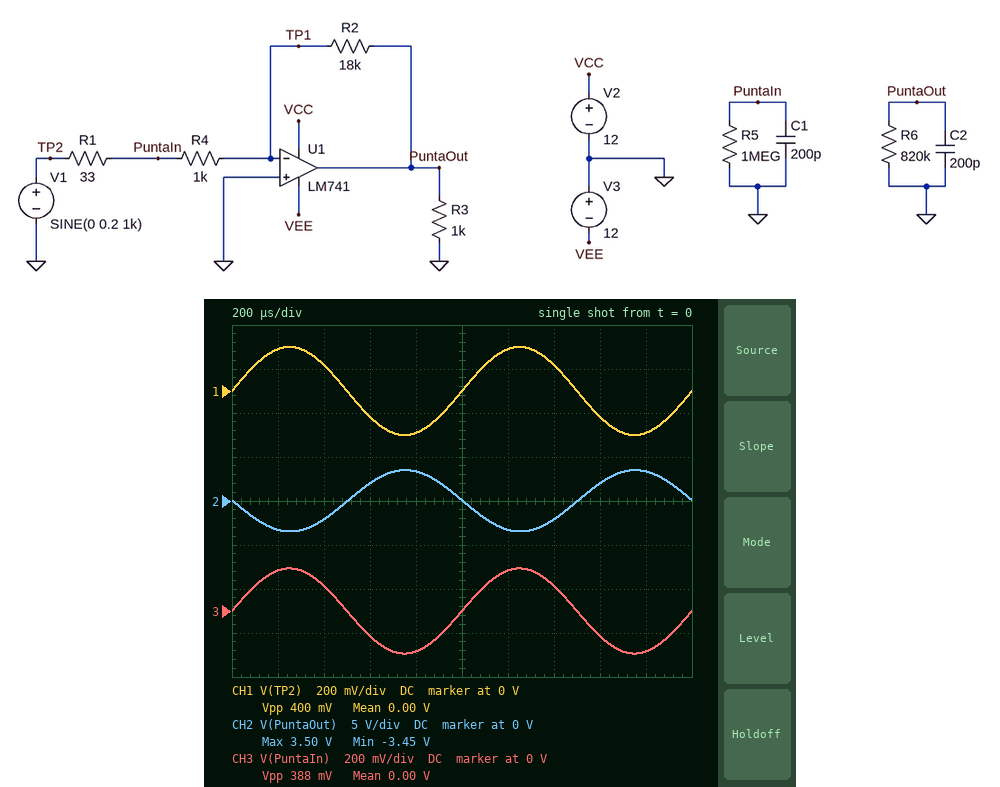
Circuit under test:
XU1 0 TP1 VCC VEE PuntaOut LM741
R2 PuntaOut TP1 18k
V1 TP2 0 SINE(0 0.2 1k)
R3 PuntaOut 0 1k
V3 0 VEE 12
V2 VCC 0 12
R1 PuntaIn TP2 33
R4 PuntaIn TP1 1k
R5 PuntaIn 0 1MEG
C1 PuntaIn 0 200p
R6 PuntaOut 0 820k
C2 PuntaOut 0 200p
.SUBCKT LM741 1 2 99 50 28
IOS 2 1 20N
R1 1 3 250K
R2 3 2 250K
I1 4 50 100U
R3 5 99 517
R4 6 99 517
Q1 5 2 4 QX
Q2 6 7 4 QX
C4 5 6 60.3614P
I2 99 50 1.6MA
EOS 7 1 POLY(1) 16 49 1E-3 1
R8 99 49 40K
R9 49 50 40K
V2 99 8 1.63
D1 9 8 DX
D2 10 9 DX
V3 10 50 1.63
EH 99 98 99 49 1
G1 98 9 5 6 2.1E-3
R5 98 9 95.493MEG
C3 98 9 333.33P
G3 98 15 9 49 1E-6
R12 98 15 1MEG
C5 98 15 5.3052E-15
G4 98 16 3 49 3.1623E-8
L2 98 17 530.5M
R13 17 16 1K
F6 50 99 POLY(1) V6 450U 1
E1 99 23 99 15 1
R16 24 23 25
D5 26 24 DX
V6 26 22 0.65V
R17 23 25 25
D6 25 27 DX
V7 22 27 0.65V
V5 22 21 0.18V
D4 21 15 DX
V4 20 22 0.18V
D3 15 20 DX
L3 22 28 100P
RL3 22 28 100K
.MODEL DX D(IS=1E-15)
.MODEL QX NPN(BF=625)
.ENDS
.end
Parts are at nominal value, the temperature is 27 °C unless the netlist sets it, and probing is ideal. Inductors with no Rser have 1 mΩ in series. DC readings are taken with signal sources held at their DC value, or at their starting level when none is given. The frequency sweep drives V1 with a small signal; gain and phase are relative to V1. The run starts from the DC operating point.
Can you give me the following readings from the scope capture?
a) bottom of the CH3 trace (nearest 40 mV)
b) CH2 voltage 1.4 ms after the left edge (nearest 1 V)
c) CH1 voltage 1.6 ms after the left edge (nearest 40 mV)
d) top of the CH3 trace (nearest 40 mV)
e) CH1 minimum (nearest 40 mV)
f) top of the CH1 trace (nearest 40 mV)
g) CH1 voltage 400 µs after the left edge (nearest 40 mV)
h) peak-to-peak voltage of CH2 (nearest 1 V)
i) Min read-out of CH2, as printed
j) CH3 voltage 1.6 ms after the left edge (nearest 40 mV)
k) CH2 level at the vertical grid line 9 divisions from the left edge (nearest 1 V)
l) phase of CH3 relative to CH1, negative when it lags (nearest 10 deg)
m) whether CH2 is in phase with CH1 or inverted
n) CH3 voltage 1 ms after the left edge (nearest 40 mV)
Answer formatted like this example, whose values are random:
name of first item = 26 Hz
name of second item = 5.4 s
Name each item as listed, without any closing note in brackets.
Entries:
bottom of the CH3 trace = -200 mV
CH2 voltage 1.4 ms after the left edge = -2 V
CH1 voltage 1.6 ms after the left edge = -120 mV
top of the CH3 trace = 200 mV
CH1 minimum = -200 mV
top of the CH1 trace = 200 mV
CH1 voltage 400 µs after the left edge = 120 mV
peak-to-peak voltage of CH2 = 7 V
Min read-out of CH2, as printed = -3.45 V
CH3 voltage 1.6 ms after the left edge = -120 mV
CH2 level at the vertical grid line 9 divisions from the left edge = 3 V
phase of CH3 relative to CH1, negative when it lags = 0 deg
whether CH2 is in phase with CH1 or inverted = inverted
CH3 voltage 1 ms after the left edge = 0 V
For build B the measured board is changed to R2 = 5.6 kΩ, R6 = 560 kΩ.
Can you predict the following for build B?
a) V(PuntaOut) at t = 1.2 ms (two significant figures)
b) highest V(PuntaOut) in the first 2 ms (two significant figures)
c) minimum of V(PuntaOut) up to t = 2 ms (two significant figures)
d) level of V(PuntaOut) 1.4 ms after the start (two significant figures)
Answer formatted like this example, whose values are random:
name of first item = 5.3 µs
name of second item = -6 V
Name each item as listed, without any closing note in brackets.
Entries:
V(PuntaOut) at t = 1.2 ms = -1.0 V
highest V(PuntaOut) in the first 2 ms = 1.1 V
minimum of V(PuntaOut) up to t = 2 ms = -1.1 V
level of V(PuntaOut) 1.4 ms after the start = -640 mV
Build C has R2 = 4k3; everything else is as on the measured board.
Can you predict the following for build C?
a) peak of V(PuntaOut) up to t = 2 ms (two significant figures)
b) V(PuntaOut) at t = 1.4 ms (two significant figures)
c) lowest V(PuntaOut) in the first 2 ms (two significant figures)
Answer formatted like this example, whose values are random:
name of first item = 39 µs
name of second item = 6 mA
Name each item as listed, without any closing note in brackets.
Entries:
peak of V(PuntaOut) up to t = 2 ms = 840 mV
V(PuntaOut) at t = 1.4 ms = -490 mV
lowest V(PuntaOut) in the first 2 ms = -830 mV
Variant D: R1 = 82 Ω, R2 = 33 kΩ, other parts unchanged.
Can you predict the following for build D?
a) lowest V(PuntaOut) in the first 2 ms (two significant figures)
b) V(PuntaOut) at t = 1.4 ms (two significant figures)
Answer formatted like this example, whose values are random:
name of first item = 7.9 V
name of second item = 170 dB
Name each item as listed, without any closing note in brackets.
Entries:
lowest V(PuntaOut) in the first 2 ms = -6.1 V
V(PuntaOut) at t = 1.4 ms = -3.7 V
